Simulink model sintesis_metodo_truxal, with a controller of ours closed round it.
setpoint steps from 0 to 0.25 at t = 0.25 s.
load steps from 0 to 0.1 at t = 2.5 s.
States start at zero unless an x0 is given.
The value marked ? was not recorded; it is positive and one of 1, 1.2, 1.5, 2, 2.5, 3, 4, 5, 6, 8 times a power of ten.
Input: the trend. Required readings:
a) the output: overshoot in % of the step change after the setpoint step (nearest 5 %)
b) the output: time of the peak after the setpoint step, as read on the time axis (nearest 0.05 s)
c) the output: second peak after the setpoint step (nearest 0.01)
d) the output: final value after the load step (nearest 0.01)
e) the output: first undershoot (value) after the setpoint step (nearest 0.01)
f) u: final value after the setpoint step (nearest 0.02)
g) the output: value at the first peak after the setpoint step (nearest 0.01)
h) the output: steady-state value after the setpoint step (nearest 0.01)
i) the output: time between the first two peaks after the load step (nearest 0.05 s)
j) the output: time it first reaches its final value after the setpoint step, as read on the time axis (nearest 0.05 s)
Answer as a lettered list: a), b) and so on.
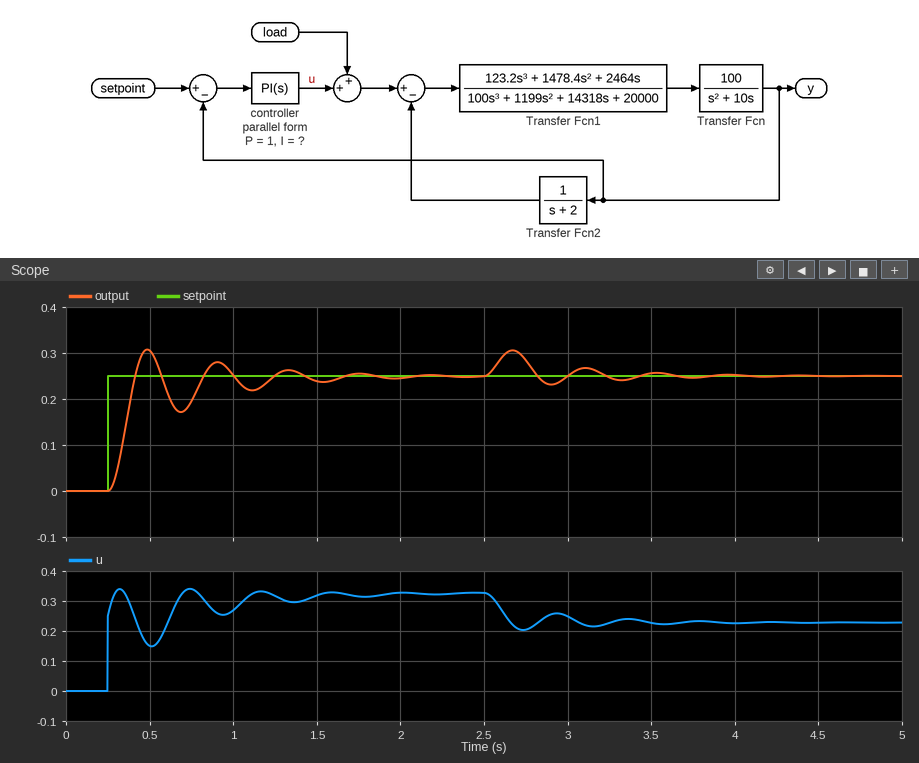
a) 25 %
b) 0.50 s
c) 0.28
d) 0.25
e) 0.17
f) 0.32
g) 0.31
h) 0.25
i) 0.45 s
j) 0.40 s
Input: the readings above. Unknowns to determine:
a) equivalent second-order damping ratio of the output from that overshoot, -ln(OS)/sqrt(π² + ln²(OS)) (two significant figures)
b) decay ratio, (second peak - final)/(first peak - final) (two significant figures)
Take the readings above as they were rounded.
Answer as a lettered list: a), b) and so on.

a) 0.40
b) 0.50
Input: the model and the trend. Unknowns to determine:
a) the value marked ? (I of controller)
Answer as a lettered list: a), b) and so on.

a) 10
